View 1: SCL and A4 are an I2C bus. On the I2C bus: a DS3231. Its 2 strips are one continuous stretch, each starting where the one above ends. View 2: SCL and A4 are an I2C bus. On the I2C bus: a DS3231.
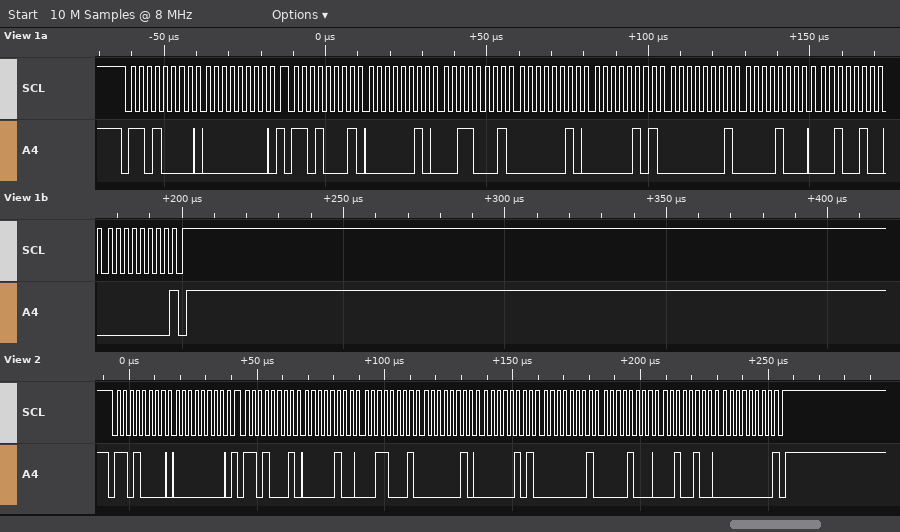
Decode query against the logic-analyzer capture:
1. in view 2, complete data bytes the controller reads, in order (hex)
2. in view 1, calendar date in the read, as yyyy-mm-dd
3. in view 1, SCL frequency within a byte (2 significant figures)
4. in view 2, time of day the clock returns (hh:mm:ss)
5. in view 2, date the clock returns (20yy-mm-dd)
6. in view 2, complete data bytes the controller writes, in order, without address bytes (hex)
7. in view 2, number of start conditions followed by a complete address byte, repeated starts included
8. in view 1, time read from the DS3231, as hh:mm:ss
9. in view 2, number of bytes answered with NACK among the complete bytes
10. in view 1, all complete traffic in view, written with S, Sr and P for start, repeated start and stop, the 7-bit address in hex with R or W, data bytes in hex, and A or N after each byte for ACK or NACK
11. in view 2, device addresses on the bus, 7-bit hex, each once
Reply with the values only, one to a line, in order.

04 31 02 05 01 08 24 00
2024-08-01
400 kHz
02:31:04
2024-08-01
00
2
02:31:02
1
S 68W A 00 A Sr 68R A 02 A 31 A 02 A 05 A 01 A 08 A 24 A 00 N P
0x68
